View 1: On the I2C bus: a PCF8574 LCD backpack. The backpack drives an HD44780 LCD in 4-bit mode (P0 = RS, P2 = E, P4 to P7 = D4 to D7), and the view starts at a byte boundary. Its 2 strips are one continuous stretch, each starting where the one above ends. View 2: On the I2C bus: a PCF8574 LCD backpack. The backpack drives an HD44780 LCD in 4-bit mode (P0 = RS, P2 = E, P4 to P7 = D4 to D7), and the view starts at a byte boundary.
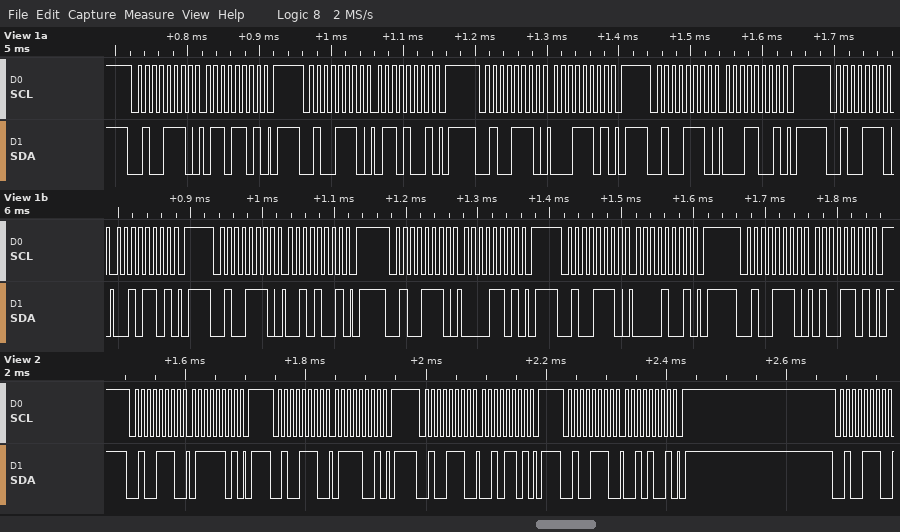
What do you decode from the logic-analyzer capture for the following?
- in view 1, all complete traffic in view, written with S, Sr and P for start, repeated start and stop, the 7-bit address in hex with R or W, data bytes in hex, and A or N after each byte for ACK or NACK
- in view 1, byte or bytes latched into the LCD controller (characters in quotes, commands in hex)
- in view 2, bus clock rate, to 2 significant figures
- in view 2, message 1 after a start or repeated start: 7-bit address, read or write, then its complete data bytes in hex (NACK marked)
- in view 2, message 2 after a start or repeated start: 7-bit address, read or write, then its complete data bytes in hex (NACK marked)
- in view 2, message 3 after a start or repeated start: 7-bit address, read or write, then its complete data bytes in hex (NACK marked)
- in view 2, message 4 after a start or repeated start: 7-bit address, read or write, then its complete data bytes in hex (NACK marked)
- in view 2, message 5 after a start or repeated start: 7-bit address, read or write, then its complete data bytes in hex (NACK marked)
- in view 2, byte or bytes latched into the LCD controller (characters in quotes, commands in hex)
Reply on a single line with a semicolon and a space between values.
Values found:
S 27W A 6D A P S 27W A 69 A P S 27W A 1D A P S 27W A 19 A P S 27W A 2D A P S 27W A 29 A P S 27W A 0D A P S 27W A 09 A P S 27W A 4D A P; 'a' ' '; 100 kHz; 0x27 write: 7D; 0x27 write: 79; 0x27 write: 2D; 0x27 write: 29; 0x27 write; 'r'
